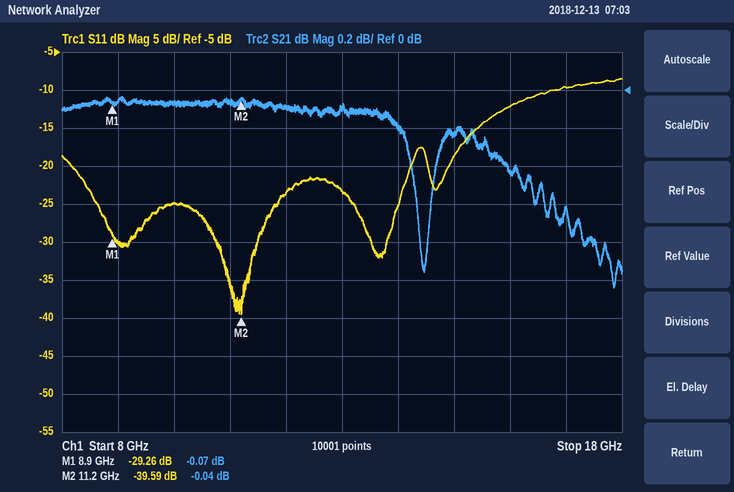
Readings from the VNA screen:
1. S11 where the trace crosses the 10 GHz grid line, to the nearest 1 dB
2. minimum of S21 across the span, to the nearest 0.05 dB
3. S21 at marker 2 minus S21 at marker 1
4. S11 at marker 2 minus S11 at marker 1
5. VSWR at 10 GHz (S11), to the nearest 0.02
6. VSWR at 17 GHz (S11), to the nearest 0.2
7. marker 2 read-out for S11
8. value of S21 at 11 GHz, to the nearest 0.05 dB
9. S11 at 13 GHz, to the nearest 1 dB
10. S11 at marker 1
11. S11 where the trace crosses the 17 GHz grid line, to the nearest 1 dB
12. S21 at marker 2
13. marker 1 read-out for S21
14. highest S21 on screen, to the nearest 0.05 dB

-25 dB
-1.05 dB
0.03 dB
-10.33 dB
1.12
2.0
-39.59 dB
-0.05 dB
-23 dB
-29.26 dB
-10 dB
-0.04 dB
-0.07 dB
-0.05 dB
